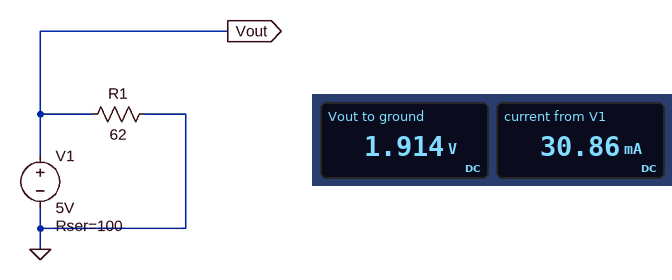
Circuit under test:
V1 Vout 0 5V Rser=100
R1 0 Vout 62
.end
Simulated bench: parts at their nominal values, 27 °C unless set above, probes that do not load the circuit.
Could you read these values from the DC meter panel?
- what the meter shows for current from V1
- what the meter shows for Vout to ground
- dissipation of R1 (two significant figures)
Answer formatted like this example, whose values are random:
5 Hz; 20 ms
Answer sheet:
30.86 mA; 1.914 V; 59 mW
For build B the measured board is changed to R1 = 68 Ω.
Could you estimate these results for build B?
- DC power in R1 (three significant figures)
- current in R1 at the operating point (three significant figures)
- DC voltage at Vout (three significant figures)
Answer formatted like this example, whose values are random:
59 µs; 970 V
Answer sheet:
60.2 mW; 29.8 mA; 2.02 V
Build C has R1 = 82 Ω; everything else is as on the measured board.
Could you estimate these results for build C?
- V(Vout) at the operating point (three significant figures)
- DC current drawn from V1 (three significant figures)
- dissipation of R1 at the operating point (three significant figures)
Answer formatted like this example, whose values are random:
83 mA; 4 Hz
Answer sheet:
2.25 V; 27.5 mA; 61.9 mW
